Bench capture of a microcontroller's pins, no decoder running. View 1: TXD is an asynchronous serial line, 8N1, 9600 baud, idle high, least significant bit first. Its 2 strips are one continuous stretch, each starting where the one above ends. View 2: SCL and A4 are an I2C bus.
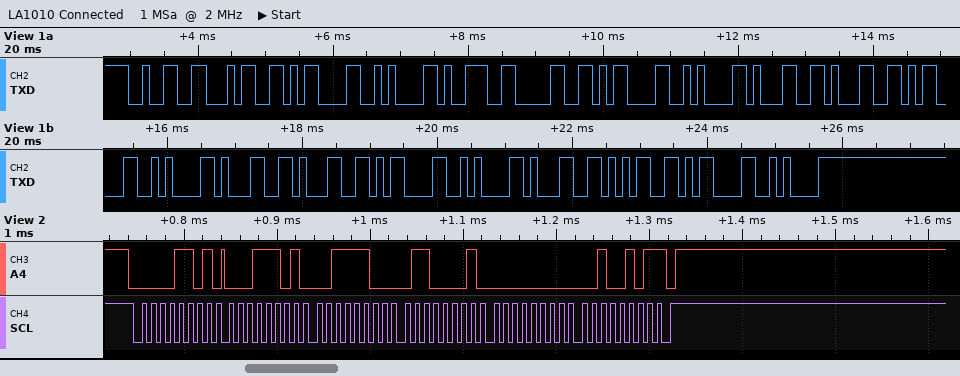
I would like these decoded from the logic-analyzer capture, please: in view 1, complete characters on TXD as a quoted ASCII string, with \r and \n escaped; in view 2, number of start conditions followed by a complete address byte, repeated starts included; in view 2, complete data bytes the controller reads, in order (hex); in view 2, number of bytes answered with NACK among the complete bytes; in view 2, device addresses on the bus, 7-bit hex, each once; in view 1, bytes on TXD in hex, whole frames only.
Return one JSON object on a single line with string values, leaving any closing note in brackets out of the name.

{"in view 1, complete characters on TXD as a quoted ASCII string, with \\r and \\n escaped": "\"24\\r\\n90\\r\\n11\\r\\n11\\r\\n15\\r\\n\"", "in view 2, number of start conditions followed by a complete address byte, repeated starts included": "1", "in view 2, complete data bytes the controller reads, in order": "1D 3C 61 00 25", "in view 2, number of bytes answered with NACK among the complete bytes": "1", "in view 2, device addresses on the bus, 7-bit hex, each once": "0x06", "in view 1, bytes on TXD in hex, whole frames only": "32 34 0D 0A 39 30 0D 0A 31 31 0D 0A 31 31 0D 0A 31 35 0D 0A"}
